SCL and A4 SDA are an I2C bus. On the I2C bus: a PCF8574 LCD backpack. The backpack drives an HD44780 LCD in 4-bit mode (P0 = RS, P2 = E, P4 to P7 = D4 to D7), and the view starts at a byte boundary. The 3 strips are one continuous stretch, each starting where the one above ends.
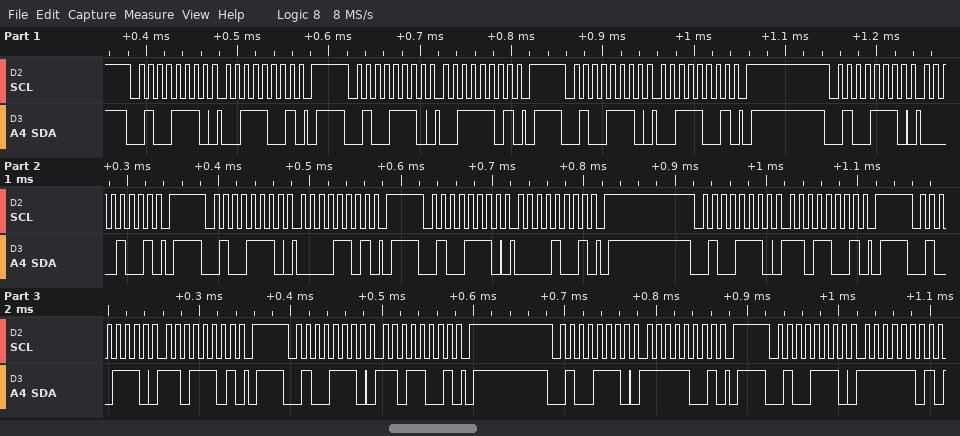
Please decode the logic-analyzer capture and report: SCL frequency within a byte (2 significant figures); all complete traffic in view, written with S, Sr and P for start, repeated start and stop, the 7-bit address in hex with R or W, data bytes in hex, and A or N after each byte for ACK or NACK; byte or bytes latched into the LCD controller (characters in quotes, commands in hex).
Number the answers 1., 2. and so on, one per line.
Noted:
1. 100 kHz
2. S 27W A 39 A P S 27W A 3D A P S 27W A 39 A P S 27W A 09 A P S 27W A 0D A P S 27W A 09 A P S 27W A D9 A P S 27W A DD A P S 27W A D9 A P S 27W A F9 A P S 27W A FD A
3. '0'
